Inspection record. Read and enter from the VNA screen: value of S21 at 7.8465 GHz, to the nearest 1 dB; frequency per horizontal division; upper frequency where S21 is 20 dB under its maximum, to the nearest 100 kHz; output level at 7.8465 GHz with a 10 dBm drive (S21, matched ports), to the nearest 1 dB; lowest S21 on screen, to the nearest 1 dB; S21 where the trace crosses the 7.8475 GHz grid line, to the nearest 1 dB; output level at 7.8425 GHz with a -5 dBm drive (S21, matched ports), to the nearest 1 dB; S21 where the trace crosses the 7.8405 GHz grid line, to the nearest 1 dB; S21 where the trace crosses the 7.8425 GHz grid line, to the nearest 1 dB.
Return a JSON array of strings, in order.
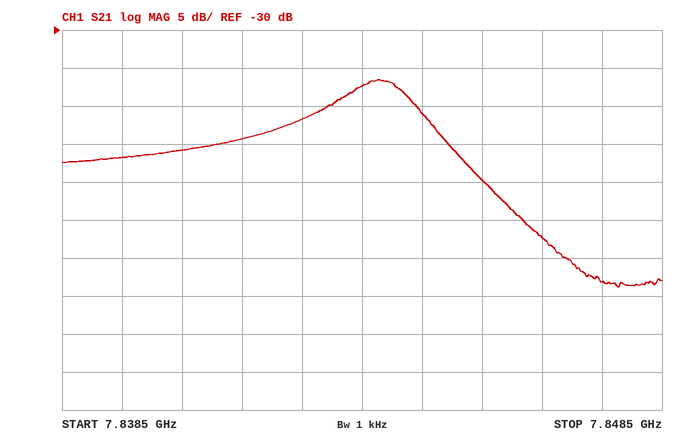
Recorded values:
["-57 dB", "1 MHz", "7.8464 GHz", "-47 dBm", "-64 dB", "-63 dB", "-47 dBm", "-46 dB", "-42 dB"]
